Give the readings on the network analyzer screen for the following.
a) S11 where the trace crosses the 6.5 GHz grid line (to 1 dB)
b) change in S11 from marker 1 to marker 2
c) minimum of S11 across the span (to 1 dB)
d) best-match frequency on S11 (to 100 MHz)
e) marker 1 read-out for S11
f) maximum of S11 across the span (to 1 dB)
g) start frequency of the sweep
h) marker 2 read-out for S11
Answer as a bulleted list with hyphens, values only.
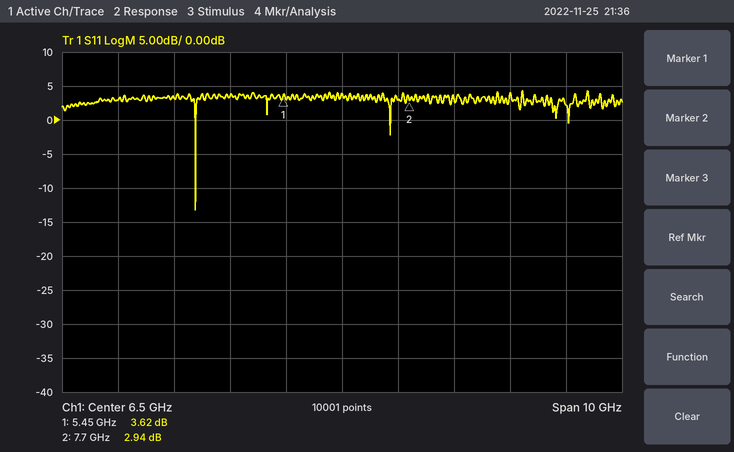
- 4 dB
- -0.68 dB
- -13 dB
- 3.9 GHz
- 3.62 dB
- 4 dB
- 1.5 GHz
- 2.94 dB
